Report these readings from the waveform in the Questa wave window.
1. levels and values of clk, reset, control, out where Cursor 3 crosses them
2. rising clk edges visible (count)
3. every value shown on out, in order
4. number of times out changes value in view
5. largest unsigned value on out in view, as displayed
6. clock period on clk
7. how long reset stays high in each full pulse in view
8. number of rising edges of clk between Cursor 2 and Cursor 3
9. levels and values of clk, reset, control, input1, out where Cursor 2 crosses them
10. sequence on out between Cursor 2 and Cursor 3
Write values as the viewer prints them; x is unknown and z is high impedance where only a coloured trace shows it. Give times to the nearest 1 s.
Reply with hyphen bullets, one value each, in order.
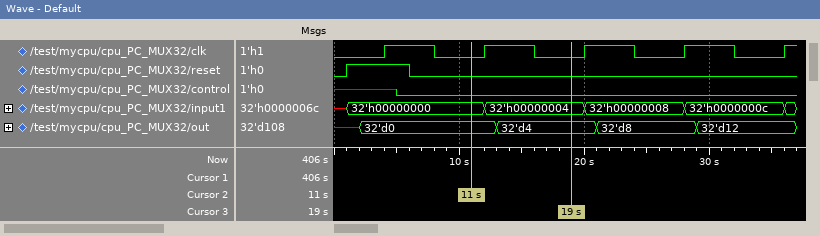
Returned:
- clk=0, reset=0, control=0, out=32'd4
- 5
- x, 32'd0, 32'd4, 32'd8, 32'd12
- 4
- 32'd12
- 8 s
- 5 s
- 1
- clk=0, reset=0, control=0, input1=32'h00000000, out=32'd0
- 32'd0, 32'd4
